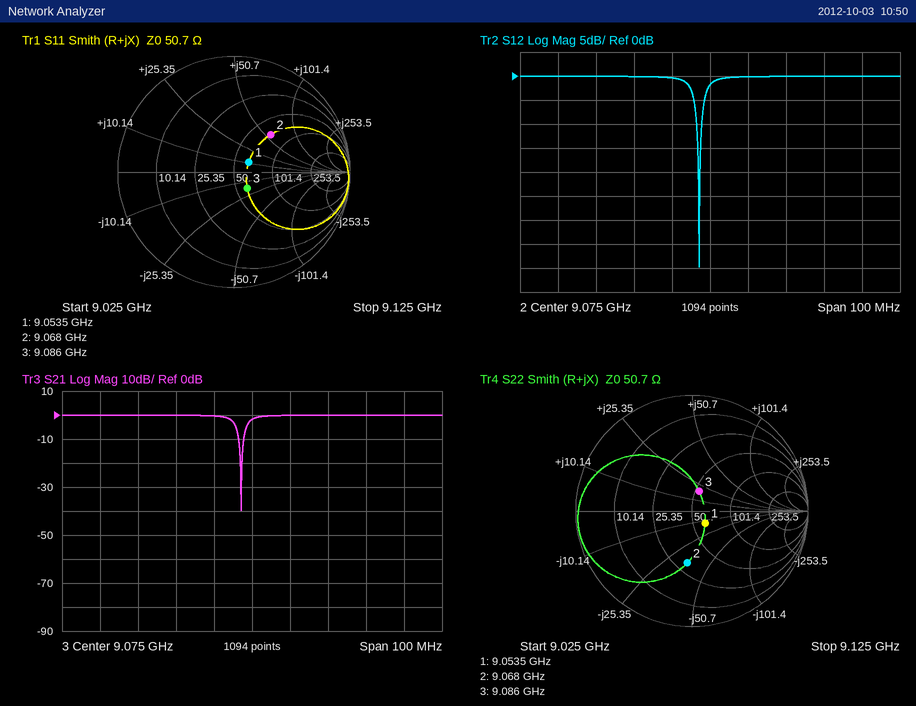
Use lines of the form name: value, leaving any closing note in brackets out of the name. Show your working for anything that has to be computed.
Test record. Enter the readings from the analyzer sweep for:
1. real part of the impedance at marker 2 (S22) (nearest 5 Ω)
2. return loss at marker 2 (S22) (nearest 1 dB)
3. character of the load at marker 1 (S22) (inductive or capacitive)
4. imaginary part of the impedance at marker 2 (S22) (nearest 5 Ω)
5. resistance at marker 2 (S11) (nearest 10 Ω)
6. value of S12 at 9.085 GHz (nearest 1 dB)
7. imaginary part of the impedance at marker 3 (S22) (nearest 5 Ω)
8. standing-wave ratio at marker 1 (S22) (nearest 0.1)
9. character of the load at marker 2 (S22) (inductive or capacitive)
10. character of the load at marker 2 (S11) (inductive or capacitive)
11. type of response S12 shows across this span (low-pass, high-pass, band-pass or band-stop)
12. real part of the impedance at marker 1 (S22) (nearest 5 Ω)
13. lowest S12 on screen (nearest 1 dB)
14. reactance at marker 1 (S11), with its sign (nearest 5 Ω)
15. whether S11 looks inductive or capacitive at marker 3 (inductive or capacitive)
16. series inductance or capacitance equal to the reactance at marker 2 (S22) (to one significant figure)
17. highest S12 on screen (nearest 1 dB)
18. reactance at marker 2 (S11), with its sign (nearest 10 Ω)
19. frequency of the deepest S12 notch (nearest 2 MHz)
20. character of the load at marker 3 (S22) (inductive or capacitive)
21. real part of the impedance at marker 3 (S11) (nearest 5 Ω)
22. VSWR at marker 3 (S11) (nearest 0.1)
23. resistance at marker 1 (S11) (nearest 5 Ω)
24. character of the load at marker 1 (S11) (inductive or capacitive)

real part of the impedance at marker 2 (S22): 30 Ω
return loss at marker 2 (S22): 7 dB
character of the load at marker 1 (S22): capacitive
imaginary part of the impedance at marker 2 (S22): -35 Ω
resistance at marker 2 (S11): 70 Ω
value of S12 at 9.085 GHz: 0 dB
imaginary part of the impedance at marker 3 (S22): +20 Ω
standing-wave ratio at marker 1 (S22): 1.4
character of the load at marker 2 (S22): capacitive
character of the load at marker 2 (S11): inductive
type of response S12 shows across this span: band-stop
real part of the impedance at marker 1 (S22): 60 Ω
lowest S12 on screen: -40 dB
reactance at marker 1 (S11), with its sign: +10 Ω
whether S11 looks inductive or capacitive at marker 3: capacitive
series inductance or capacitance equal to the reactance at marker 2 (S22): C = 1/(2π × 9.068 GHz × 35 Ω) ≈ 501 fF, so 500 fF to one significant figure
highest S12 on screen: 0 dB
reactance at marker 2 (S11), with its sign: +60 Ω
frequency of the deepest S12 notch: 9.072 GHz
character of the load at marker 3 (S22): inductive
real part of the impedance at marker 3 (S11): 60 Ω
VSWR at marker 3 (S11): 1.4
resistance at marker 1 (S11): 65 Ω
character of the load at marker 1 (S11): inductive
